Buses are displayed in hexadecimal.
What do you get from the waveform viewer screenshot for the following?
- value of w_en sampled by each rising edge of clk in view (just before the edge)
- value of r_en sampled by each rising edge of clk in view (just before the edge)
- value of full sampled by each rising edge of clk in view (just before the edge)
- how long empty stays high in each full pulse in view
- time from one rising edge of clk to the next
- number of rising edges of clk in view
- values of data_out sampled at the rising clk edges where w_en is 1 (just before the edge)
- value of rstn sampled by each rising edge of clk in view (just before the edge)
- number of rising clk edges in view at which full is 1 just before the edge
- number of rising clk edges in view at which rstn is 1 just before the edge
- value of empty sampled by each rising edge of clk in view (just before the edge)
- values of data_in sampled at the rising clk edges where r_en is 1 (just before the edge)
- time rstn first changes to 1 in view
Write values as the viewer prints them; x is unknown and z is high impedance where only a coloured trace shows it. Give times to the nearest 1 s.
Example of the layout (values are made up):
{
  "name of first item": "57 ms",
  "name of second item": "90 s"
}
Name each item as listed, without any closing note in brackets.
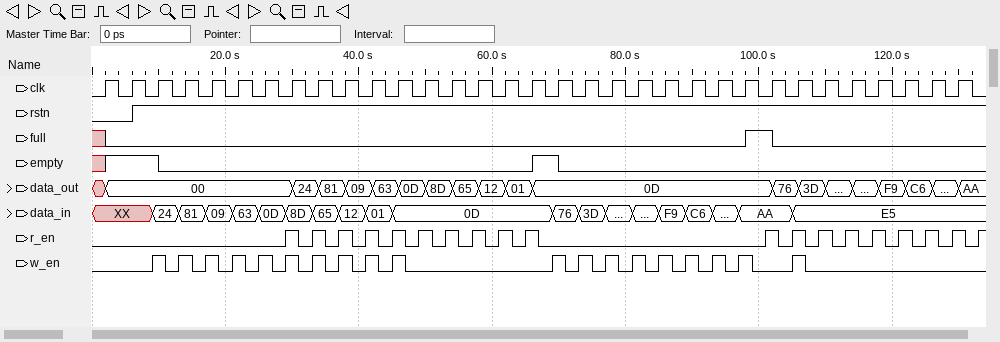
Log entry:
{
  "value of w_en sampled by each rising edge of clk in view": "0 0 1 1 1 1 1 1 1 1 1 1 0 0 0 0 0 1 1 1 1 1 1 1 1 0 1 0 0 0 0 0 0",
  "value of r_en sampled by each rising edge of clk in view": "0 0 0 0 0 0 0 1 1 1 1 1 1 1 1 1 1 0 0 0 0 0 0 0 0 1 1 1 1 1 1 1 1",
  "value of full sampled by each rising edge of clk in view": "x 0 0 0 0 0 0 0 0 0 0 0 0 0 0 0 0 0 0 0 0 0 0 0 0 1 0 0 0 0 0 0 0",
  "how long empty stays high in each full pulse in view": "4 s",
  "time from one rising edge of clk to the next": "4 s",
  "number of rising edges of clk in view": "33",
  "values of data_out sampled at the rising clk edges where w_en is 1": "00, 00, 00, 00, 00, 00, 24, 81, 09, 63, 0D, 0D, 0D, 0D, 0D, 0D, 0D, 0D, 76",
  "value of rstn sampled by each rising edge of clk in view": "0 0 1 1 1 1 1 1 1 1 1 1 1 1 1 1 1 1 1 1 1 1 1 1 1 1 1 1 1 1 1 1 1",
  "number of rising clk edges in view at which full is 1 just before the edge": "1",
  "number of rising clk edges in view at which rstn is 1 just before the edge": "31",
  "value of empty sampled by each rising edge of clk in view": "x 1 1 0 0 0 0 0 0 0 0 0 0 0 0 0 0 1 0 0 0 0 0 0 0 0 0 0 0 0 0 0 0",
  "values of data_in sampled at the rising clk edges where r_en is 1": "8D, 65, 12, 01, 0D, 0D, 0D, 0D, 0D, 0D, AA, E5, E5, E5, E5, E5, E5, E5",
  "time rstn first changes to 1 in view": "6 s"
}
